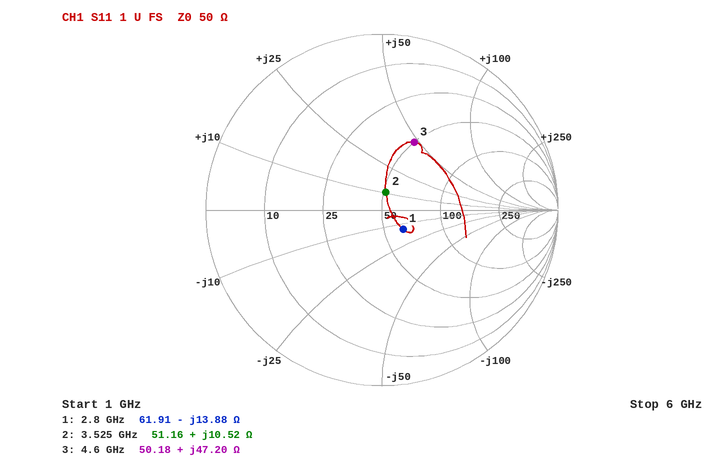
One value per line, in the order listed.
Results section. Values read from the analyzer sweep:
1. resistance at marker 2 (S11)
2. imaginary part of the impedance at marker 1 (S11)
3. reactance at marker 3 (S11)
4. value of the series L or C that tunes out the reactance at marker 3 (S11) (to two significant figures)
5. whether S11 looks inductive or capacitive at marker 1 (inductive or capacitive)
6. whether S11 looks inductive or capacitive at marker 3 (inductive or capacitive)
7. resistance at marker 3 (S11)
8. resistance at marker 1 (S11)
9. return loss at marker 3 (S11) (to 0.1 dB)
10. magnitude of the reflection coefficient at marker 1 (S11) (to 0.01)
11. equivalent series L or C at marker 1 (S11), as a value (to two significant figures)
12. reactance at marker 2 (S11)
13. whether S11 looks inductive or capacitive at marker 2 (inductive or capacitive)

51.16 Ω
-13.88 Ω
+47.20 Ω
730 fF
capacitive
inductive
50.18 Ω
61.91 Ω
7.4 dB
0.16
4.1 pF
+10.52 Ω
inductive
